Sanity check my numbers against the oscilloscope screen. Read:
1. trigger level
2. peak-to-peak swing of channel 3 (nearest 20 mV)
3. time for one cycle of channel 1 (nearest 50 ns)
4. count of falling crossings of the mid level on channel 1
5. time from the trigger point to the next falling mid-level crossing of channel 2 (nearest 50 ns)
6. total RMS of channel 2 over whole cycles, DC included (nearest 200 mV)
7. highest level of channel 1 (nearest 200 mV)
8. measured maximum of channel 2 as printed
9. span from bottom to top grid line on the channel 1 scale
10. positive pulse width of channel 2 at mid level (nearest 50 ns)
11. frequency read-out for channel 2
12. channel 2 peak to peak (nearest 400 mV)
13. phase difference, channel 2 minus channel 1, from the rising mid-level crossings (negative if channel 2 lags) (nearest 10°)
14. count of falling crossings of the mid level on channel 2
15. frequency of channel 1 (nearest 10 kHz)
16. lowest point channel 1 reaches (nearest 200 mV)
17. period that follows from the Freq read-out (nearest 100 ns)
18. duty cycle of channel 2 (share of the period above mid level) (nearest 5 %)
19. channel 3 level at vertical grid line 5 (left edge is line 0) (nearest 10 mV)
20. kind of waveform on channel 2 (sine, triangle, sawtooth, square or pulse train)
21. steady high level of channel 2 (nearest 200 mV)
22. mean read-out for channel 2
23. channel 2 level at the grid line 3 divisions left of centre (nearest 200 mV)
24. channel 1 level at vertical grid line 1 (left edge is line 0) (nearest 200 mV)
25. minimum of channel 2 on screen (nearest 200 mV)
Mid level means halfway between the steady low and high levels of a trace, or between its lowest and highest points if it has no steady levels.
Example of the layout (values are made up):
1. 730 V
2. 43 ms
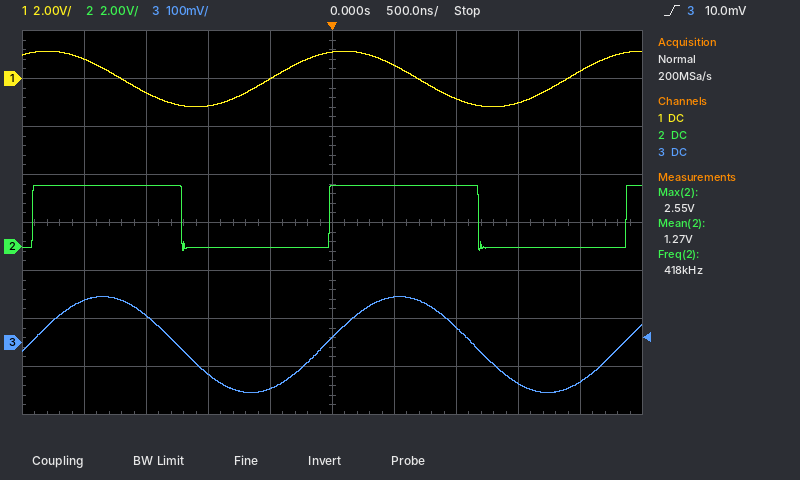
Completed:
1. 10.0 mV
2. 200 mV
3. 2.40 µs
4. 2
5. 1.20 µs
6. 1.8 V
7. 1.2 V
8. 2.55 V
9. 16 V
10. 1.20 µs
11. 418 kHz
12. 2.8 V
13. -70°
14. 2
15. 420 kHz
16. -1.2 V
17. 2.4 µs
18. 50 %
19. 10 mV
20. square
21. 2.6 V
22. 1.27 V
23. 2.6 V
24. 800 mV
25. -200 mV
